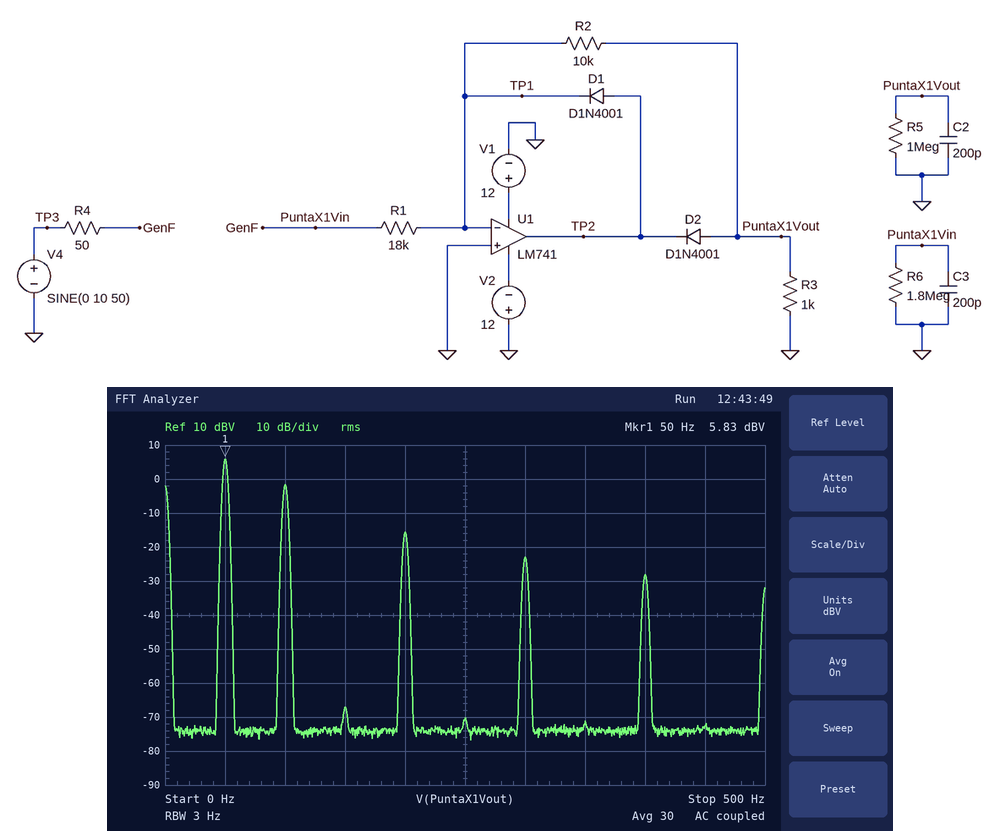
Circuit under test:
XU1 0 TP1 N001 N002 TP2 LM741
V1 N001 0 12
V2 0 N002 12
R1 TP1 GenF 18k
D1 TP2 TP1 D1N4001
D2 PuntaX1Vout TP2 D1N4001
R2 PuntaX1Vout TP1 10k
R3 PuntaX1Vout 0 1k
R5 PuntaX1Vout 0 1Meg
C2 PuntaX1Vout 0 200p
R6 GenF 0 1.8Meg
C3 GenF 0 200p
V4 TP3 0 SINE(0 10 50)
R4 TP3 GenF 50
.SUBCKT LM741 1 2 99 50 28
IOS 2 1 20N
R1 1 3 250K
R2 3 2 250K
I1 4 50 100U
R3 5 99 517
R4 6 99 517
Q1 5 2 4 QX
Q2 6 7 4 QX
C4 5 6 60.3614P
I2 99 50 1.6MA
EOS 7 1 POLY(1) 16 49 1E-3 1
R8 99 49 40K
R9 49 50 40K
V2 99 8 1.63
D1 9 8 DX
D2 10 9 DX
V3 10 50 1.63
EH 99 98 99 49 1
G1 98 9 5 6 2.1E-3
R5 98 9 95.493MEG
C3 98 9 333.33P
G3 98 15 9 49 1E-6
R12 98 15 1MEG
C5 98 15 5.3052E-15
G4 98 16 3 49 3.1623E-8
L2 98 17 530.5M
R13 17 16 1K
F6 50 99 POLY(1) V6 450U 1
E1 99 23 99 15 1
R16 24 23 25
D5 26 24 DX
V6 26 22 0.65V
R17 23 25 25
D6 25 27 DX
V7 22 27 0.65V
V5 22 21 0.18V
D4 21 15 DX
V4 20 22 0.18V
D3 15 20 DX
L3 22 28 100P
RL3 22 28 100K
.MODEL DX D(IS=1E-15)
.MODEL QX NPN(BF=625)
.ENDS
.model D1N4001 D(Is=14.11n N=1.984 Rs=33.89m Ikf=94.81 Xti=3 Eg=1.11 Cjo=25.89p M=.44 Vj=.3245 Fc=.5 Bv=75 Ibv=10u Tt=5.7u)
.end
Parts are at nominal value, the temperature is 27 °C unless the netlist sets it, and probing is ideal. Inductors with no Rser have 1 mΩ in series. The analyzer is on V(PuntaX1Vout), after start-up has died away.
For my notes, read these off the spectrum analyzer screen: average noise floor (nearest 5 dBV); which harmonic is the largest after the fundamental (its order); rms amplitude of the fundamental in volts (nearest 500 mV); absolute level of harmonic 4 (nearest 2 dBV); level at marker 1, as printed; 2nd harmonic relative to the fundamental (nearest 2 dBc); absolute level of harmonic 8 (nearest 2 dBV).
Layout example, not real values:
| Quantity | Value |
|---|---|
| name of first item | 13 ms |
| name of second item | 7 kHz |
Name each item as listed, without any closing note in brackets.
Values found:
| Quantity | Value |
|---|---|
| average noise floor | -75 dBV |
| which harmonic is the largest after the fundamental | 2 |
| rms amplitude of the fundamental in volts | 2.0 V |
| absolute level of harmonic 4 | -16 dBV |
| level at marker 1, as printed | 5.83 dBV |
| 2nd harmonic relative to the fundamental | -8 dBc |
| absolute level of harmonic 8 | -28 dBV |
